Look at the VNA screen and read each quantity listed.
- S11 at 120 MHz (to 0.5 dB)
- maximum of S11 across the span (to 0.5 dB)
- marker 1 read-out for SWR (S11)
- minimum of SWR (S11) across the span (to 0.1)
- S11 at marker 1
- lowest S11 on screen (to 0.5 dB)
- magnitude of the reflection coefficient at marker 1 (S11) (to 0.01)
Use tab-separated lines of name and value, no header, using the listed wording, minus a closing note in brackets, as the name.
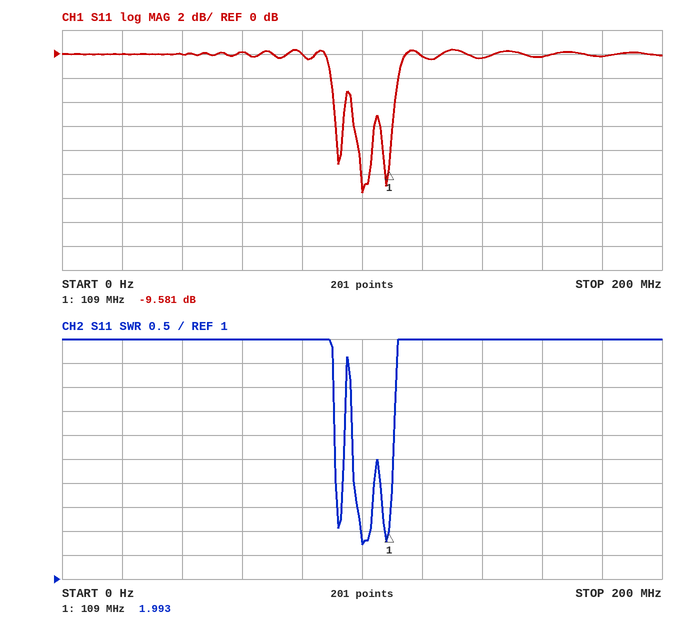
S11 at 120 MHz	0.0 dB
maximum of S11 across the span	0.5 dB
marker 1 read-out for SWR	1.993
minimum of SWR (S11) across the span	1.7
S11 at marker 1	-9.581 dB
lowest S11 on screen	-11.5 dB
magnitude of the reflection coefficient at marker 1 (S11)	0.33
